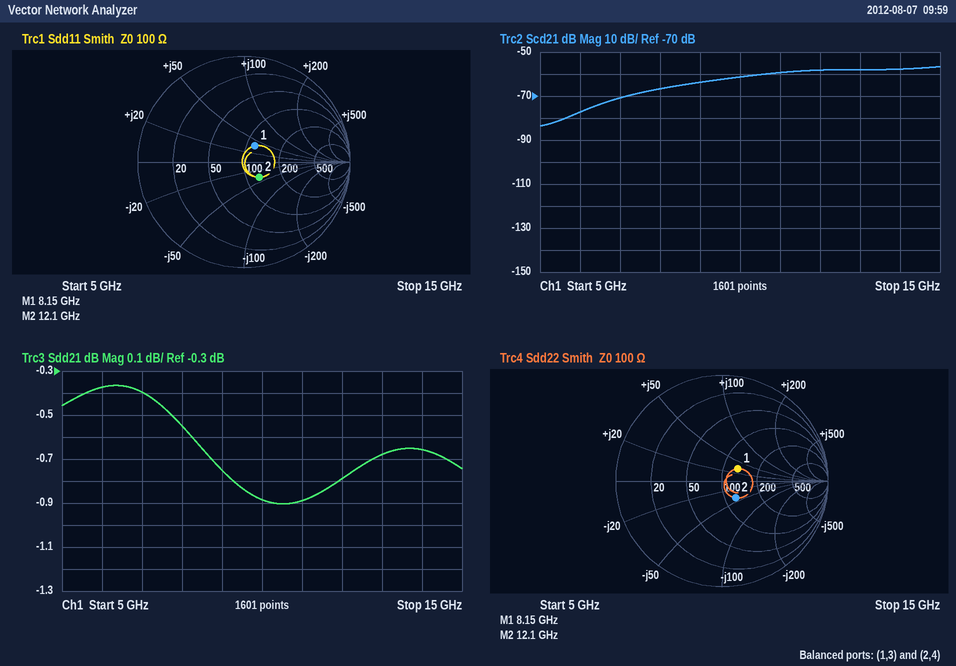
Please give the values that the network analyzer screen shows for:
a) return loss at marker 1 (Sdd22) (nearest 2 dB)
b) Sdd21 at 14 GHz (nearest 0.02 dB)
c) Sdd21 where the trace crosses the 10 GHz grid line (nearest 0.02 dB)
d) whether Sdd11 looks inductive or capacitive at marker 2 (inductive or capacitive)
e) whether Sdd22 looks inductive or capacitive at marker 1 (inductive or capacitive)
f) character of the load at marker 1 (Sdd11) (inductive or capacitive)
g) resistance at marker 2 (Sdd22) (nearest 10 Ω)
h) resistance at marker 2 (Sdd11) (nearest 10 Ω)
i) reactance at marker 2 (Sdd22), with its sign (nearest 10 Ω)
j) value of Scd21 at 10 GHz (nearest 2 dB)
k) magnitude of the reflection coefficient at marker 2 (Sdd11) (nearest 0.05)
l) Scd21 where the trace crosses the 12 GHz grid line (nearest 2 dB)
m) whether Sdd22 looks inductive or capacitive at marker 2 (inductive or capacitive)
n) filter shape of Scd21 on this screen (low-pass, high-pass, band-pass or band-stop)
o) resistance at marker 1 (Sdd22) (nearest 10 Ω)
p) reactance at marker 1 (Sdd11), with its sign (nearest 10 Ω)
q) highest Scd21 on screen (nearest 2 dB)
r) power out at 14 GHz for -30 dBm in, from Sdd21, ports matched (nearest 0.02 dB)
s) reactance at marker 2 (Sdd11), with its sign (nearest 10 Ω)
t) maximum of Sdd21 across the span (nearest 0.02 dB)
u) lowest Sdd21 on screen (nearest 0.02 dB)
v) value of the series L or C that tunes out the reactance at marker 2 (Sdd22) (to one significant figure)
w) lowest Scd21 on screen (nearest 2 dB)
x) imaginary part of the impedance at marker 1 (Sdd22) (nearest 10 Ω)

14 dB
-0.66 dB
-0.88 dB
capacitive
inductive
inductive
120 Ω
130 Ω
-40 Ω
-62 dB
0.20
-58 dB
capacitive
high-pass
130 Ω
+40 Ω
-56 dB
-30.66 dBm
-40 Ω
-0.36 dB
-0.90 dB
500 pH
-84 dB
+30 Ω
